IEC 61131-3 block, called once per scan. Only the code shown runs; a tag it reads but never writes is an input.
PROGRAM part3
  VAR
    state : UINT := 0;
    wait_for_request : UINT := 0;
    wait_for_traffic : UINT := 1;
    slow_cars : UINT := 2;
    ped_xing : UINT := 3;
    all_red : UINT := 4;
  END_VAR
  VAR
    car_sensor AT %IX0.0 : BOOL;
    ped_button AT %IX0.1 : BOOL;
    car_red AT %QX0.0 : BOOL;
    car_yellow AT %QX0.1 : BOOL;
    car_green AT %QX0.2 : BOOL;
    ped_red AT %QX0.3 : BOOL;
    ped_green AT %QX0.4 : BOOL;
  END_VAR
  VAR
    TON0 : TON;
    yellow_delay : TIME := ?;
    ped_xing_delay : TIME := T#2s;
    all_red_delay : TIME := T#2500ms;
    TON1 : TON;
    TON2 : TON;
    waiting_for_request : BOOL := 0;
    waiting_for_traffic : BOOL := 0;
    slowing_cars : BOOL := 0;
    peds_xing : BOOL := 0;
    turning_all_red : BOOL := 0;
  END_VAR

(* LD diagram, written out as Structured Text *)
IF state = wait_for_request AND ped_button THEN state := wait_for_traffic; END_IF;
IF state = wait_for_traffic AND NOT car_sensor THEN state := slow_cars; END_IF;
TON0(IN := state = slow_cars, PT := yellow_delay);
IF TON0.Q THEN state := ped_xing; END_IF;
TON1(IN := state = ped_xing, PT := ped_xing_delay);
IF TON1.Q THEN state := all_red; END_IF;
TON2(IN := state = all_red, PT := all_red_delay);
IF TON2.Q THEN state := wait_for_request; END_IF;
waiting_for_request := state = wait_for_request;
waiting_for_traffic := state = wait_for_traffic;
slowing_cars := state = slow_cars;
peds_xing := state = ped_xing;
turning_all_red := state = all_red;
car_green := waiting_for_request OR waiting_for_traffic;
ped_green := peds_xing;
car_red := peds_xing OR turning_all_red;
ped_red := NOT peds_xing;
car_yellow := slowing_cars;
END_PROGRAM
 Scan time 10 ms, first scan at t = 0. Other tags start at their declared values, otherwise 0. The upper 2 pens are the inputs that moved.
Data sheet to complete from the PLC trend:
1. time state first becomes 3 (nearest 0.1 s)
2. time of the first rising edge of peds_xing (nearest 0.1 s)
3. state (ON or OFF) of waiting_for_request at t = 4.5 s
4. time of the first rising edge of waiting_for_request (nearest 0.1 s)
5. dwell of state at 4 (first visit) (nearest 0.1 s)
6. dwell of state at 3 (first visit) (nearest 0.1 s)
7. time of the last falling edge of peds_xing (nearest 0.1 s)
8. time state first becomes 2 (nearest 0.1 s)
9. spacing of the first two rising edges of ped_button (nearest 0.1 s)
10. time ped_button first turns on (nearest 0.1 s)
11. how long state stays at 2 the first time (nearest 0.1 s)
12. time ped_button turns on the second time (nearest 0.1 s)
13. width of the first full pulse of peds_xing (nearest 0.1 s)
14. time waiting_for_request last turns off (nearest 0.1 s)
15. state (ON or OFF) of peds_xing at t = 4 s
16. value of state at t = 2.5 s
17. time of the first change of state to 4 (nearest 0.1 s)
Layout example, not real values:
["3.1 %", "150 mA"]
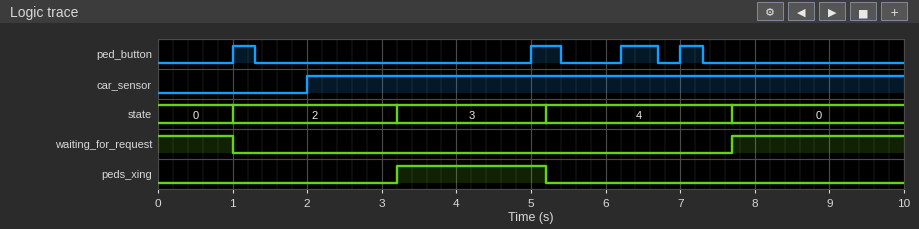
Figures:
["3.2 s", "3.2 s", "OFF", "7.7 s", "2.5 s", "2.0 s", "5.2 s", "1.0 s", "4.0 s", "1.0 s", "2.2 s", "5.0 s", "2.0 s", "1.0 s", "ON", "2", "5.2 s"]
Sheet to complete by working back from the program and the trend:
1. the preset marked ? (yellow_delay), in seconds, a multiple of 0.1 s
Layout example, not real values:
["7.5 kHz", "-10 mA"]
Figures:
["2.2 s"]
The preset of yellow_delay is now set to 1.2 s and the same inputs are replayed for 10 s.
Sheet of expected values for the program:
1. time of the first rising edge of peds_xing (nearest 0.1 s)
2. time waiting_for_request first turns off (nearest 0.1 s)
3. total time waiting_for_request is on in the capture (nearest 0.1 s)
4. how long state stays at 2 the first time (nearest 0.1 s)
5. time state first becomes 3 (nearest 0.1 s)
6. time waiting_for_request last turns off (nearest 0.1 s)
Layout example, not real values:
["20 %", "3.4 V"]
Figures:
["2.2 s", "1.0 s", "1.3 s", "1.2 s", "2.2 s", "7.0 s"]
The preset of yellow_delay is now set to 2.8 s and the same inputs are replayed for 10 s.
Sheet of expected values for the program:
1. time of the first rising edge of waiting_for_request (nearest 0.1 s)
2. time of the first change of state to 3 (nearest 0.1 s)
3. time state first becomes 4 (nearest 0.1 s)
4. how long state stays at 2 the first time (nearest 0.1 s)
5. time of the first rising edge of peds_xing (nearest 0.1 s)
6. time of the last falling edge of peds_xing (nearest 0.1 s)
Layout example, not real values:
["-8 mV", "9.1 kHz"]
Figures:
["8.3 s", "3.8 s", "5.8 s", "2.8 s", "3.8 s", "5.8 s"]
